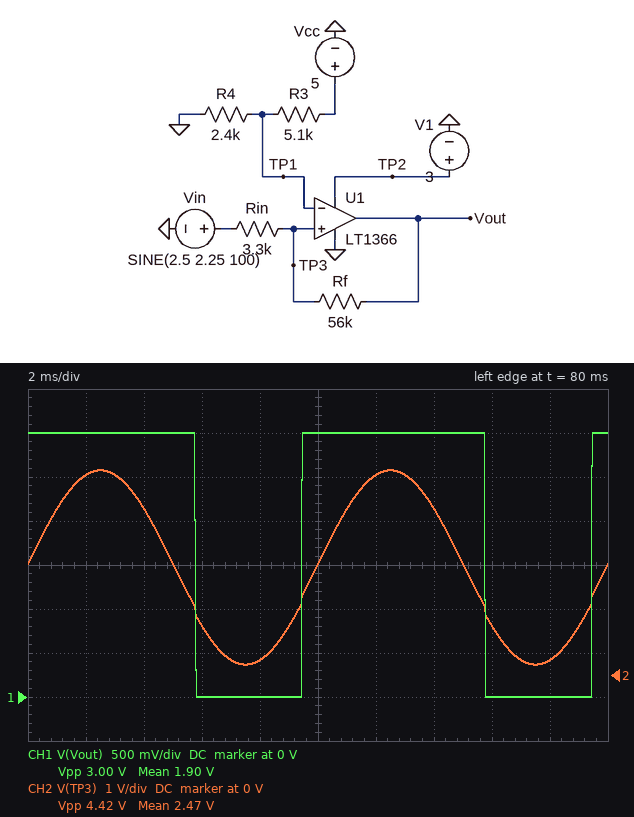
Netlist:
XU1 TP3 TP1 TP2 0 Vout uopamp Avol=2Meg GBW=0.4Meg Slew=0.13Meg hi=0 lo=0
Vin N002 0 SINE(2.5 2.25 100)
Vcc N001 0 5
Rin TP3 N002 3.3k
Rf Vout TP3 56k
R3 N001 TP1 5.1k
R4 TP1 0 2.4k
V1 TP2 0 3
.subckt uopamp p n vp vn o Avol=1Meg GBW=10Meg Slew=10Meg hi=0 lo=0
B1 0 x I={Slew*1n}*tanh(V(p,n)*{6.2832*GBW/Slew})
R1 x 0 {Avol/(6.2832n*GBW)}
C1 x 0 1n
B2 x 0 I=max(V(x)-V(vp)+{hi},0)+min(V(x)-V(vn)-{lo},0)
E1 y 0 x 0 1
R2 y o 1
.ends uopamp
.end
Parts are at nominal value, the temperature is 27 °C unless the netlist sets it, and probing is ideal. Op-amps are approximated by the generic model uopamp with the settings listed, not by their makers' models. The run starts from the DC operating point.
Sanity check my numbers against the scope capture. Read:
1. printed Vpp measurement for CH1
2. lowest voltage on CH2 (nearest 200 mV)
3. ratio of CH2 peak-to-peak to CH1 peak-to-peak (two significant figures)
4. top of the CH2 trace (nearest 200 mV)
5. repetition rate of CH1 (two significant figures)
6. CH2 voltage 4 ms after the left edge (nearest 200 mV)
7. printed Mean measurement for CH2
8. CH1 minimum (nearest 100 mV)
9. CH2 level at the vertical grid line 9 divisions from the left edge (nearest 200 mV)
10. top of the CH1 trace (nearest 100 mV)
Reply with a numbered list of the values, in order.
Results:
1. 3.00 V
2. 200 mV
3. 1.5
4. 4.6 V
5. 100 Hz
6. 3.8 V
7. 2.47 V
8. 0 V
9. 400 mV
10. 3.0 V
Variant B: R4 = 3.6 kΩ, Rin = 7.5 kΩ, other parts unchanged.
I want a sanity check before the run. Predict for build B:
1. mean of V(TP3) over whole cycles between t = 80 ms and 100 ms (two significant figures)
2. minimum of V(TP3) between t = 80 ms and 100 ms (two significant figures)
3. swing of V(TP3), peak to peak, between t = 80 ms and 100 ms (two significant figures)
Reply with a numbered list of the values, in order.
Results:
1. 2.4 V
2. 220 mV
3. 4.3 V
